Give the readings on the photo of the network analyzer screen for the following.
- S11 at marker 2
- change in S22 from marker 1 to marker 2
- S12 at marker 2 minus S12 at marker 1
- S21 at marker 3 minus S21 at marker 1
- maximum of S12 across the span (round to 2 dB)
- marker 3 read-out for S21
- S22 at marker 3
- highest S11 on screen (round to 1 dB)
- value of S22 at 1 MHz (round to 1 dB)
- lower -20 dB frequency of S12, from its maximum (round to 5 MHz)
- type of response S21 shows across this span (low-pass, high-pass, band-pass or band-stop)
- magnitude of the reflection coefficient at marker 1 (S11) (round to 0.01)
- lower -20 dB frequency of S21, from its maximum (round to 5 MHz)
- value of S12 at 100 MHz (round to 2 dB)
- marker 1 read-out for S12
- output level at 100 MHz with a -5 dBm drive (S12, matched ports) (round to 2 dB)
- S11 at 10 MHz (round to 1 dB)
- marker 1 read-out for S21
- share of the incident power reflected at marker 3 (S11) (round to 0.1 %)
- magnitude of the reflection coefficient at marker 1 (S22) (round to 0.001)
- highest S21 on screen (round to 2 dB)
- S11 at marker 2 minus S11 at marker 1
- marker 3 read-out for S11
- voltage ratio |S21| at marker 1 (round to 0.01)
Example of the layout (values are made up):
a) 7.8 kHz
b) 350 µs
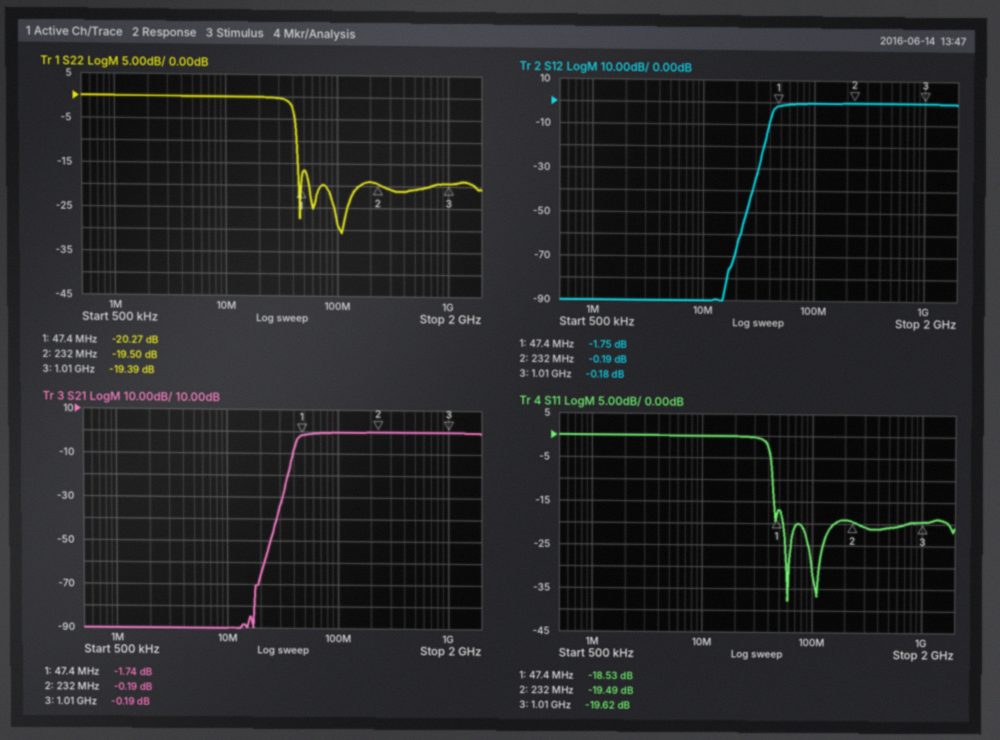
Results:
a) -19.49 dB
b) 0.77 dB
c) 1.56 dB
d) 1.55 dB
e) 0 dB
f) -0.19 dB
g) -19.39 dB
h) 0 dB
i) 0 dB
j) 35 MHz
k) high-pass
l) 0.12
m) 35 MHz
n) 0 dB
o) -1.75 dB
p) -6 dBm
q) 0 dB
r) -1.74 dB
s) 1.1 %
t) 0.097
u) 0 dB
v) -0.96 dB
w) -19.62 dB
x) 0.82
